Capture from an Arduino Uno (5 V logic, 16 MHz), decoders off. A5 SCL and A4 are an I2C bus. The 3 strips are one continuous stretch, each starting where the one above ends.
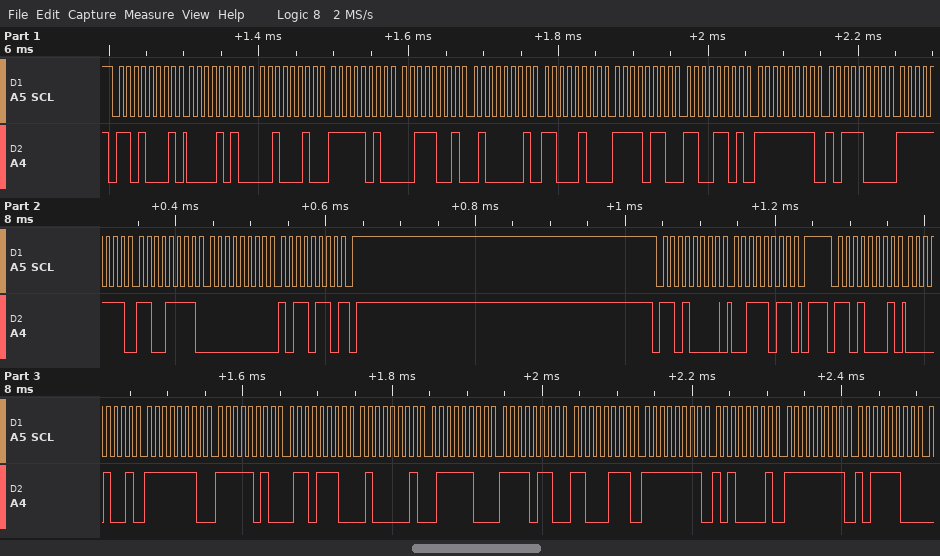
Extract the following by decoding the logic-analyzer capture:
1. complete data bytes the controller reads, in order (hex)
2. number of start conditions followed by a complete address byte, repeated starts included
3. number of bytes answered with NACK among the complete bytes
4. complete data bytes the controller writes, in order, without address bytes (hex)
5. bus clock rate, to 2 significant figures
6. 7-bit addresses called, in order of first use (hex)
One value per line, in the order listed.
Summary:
0A 22 FA 39 41 C4 F6 CD FF B8 FF CF 00 B6 09 FE FA 6E 41 7C F6 C7 FF A1 FF BC
3
1
3B
100 kHz
0x68
